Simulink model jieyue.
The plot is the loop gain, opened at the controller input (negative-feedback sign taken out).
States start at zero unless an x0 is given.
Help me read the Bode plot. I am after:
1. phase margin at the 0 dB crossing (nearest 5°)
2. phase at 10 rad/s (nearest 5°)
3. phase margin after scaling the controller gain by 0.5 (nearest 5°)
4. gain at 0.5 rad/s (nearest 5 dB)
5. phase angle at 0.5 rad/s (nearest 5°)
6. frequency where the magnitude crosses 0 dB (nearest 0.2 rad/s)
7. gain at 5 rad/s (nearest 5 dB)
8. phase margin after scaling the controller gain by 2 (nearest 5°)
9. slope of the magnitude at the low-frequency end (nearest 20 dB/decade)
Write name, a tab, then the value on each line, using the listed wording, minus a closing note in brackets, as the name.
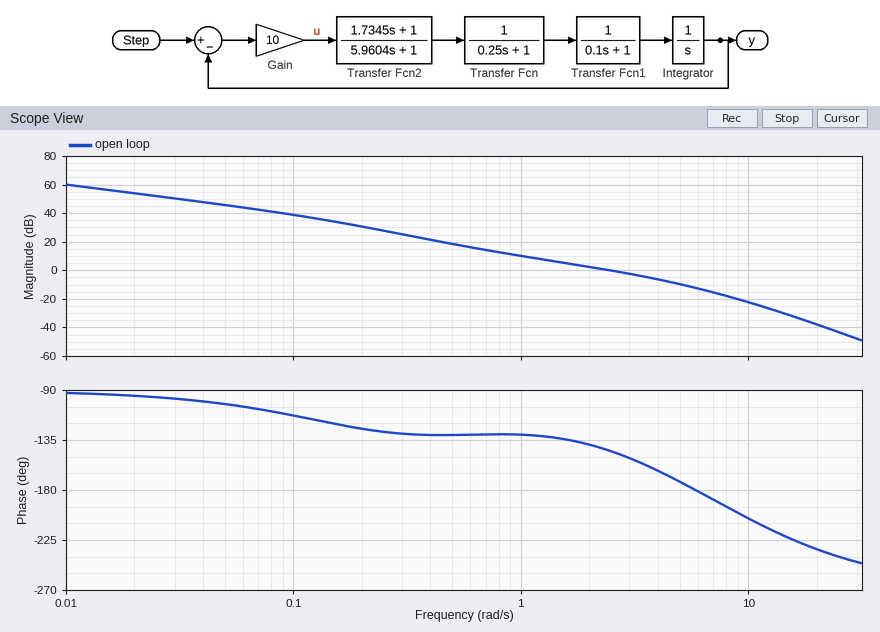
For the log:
phase margin at the 0 dB crossing	35°
phase at 10 rad/s	-205°
phase margin after scaling the controller gain by 0.5	45°
gain at 0.5 rad/s	20 dB
phase angle at 0.5 rad/s	-130°
frequency where the magnitude crosses 0 dB	2.4 rad/s
gain at 5 rad/s	-10 dB
phase margin after scaling the controller gain by 2	20°
slope of the magnitude at the low-frequency end	-20 dB/decade
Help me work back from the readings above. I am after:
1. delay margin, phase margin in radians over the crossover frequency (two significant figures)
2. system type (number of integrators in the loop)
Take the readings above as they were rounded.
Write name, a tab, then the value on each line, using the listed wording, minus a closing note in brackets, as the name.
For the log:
delay margin, phase margin in radians over the crossover frequency	0.25 s
system type	1
